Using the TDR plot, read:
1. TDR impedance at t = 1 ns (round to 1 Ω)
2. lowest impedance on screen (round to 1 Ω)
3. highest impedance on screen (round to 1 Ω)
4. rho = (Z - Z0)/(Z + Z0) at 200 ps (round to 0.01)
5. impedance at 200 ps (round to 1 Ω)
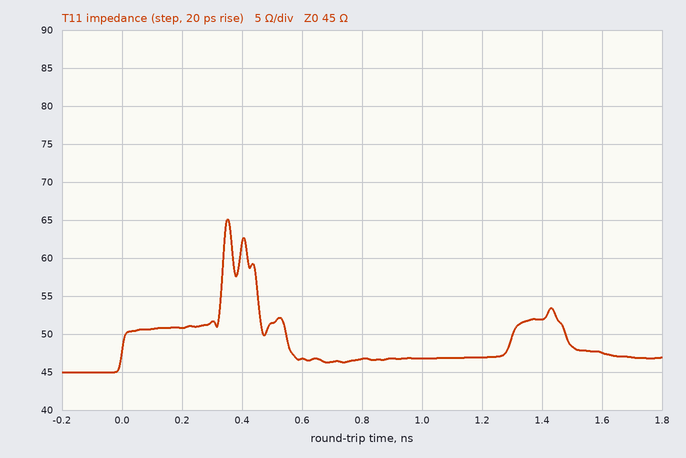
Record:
47 Ω
45 Ω
65 Ω
+0.06
51 Ω
